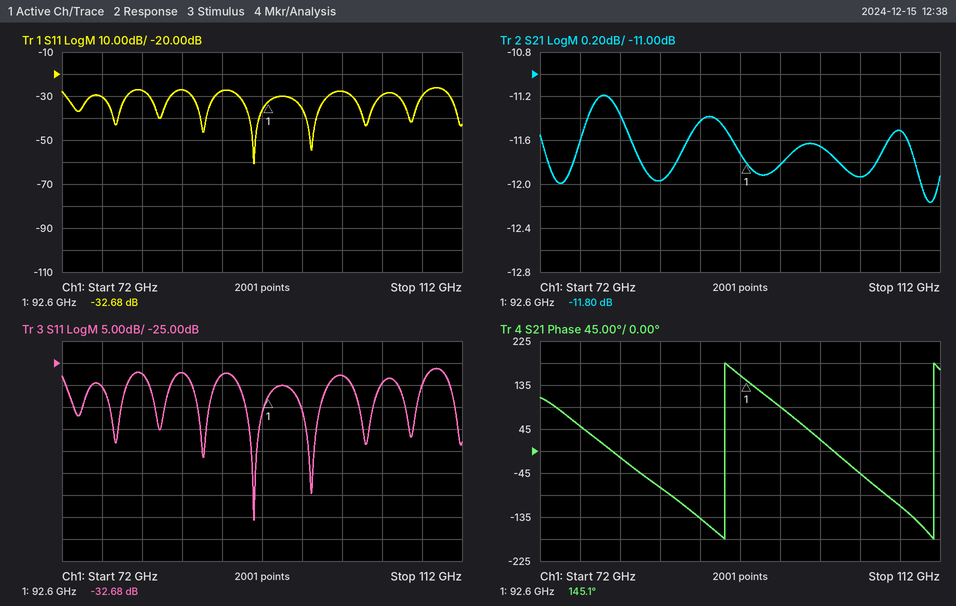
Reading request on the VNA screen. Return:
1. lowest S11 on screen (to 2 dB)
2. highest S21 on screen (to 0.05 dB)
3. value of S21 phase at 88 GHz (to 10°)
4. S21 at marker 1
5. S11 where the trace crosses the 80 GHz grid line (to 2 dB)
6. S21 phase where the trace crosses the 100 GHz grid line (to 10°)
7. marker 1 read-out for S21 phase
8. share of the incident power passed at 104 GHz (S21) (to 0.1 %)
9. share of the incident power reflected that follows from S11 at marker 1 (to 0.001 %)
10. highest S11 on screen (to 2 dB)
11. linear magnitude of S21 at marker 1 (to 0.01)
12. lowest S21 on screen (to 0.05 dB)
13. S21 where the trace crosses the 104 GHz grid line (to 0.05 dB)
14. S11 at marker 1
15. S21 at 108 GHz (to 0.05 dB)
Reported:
-60 dB
-11.20 dB
-140°
-11.80 dB
-28 dB
20°
145.1°
6.4 %
0.054 %
-26 dB
0.26
-12.15 dB
-11.95 dB
-32.68 dB
-11.50 dB
